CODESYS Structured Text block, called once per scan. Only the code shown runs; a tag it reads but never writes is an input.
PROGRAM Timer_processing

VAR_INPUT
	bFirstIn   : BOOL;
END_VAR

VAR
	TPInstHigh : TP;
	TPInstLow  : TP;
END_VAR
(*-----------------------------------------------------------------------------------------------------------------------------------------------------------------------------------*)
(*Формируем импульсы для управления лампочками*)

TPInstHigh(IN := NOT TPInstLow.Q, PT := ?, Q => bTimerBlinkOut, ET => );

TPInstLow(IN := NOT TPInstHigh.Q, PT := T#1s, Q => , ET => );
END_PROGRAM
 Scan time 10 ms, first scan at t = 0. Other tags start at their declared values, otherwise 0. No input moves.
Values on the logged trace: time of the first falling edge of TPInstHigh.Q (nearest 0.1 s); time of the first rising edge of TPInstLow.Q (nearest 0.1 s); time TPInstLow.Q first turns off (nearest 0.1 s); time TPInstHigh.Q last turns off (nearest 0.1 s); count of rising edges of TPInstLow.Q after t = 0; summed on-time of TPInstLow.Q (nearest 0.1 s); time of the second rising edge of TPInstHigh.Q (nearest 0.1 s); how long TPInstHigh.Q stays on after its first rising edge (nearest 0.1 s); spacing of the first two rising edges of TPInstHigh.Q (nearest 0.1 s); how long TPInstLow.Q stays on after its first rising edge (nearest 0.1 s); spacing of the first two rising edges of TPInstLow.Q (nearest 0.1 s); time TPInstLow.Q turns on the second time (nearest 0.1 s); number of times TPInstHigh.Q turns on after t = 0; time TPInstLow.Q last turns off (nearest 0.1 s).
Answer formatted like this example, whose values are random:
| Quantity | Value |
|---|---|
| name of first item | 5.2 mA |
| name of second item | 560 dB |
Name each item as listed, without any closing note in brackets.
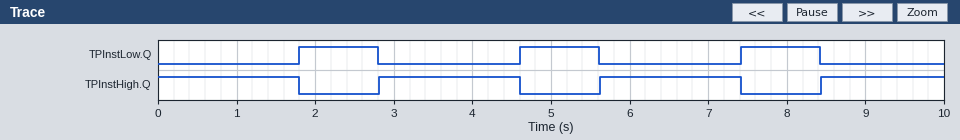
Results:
| Quantity | Value |
|---|---|
| time of the first falling edge of TPInstHigh.Q | 1.8 s |
| time of the first rising edge of TPInstLow.Q | 1.8 s |
| time TPInstLow.Q first turns off | 2.8 s |
| time TPInstHigh.Q last turns off | 7.4 s |
| count of rising edges of TPInstLow.Q after t = 0 | 3 |
| summed on-time of TPInstLow.Q | 3.0 s |
| time of the second rising edge of TPInstHigh.Q | 5.6 s |
| how long TPInstHigh.Q stays on after its first rising edge | 1.8 s |
| spacing of the first two rising edges of TPInstHigh.Q | 2.8 s |
| how long TPInstLow.Q stays on after its first rising edge | 1.0 s |
| spacing of the first two rising edges of TPInstLow.Q | 2.8 s |
| time TPInstLow.Q turns on the second time | 4.6 s |
| number of times TPInstHigh.Q turns on after t = 0 | 3 |
| time TPInstLow.Q last turns off | 8.4 s |
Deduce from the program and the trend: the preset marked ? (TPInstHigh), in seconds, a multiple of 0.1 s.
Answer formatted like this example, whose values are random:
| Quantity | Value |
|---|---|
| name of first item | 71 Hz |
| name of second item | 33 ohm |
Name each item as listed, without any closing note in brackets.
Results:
| Quantity | Value |
|---|---|
| the preset marked ? (TPInstHigh), in seconds, a multiple of 0.1 s | 1.8 s |
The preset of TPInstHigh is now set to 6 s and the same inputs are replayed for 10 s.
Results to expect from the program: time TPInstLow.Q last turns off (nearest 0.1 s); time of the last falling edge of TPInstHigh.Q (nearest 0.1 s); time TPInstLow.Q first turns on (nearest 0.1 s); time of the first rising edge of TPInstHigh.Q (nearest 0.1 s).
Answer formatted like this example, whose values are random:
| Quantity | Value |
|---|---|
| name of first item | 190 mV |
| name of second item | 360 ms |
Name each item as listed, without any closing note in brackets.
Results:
| Quantity | Value |
|---|---|
| time TPInstLow.Q last turns off | 7.0 s |
| time of the last falling edge of TPInstHigh.Q | 6.0 s |
| time TPInstLow.Q first turns on | 6.0 s |
| time of the first rising edge of TPInstHigh.Q | 7.0 s |
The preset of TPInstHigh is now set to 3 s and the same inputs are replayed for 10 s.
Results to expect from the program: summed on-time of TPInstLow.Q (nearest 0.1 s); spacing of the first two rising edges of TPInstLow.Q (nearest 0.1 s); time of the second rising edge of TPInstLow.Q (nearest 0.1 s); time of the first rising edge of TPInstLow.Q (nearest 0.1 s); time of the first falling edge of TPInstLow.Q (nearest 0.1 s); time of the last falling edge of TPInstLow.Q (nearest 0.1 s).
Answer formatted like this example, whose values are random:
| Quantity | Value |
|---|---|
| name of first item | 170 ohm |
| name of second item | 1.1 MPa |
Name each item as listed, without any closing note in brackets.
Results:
| Quantity | Value |
|---|---|
| summed on-time of TPInstLow.Q | 2.0 s |
| spacing of the first two rising edges of TPInstLow.Q | 4.0 s |
| time of the second rising edge of TPInstLow.Q | 7.0 s |
| time of the first rising edge of TPInstLow.Q | 3.0 s |
| time of the first falling edge of TPInstLow.Q | 4.0 s |
| time of the last falling edge of TPInstLow.Q | 8.0 s |
